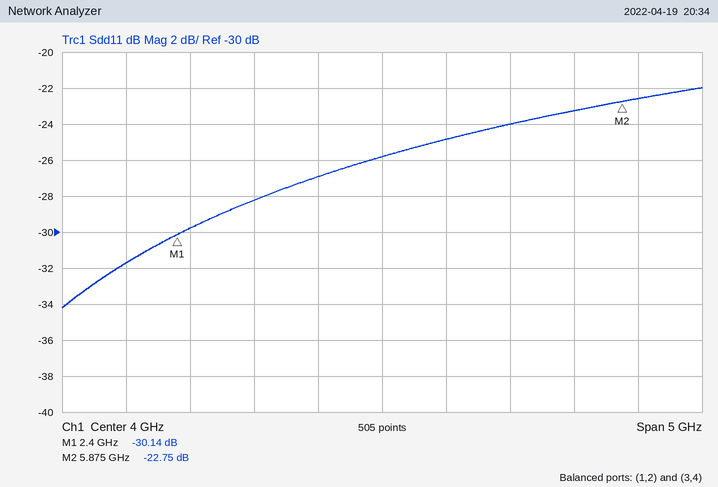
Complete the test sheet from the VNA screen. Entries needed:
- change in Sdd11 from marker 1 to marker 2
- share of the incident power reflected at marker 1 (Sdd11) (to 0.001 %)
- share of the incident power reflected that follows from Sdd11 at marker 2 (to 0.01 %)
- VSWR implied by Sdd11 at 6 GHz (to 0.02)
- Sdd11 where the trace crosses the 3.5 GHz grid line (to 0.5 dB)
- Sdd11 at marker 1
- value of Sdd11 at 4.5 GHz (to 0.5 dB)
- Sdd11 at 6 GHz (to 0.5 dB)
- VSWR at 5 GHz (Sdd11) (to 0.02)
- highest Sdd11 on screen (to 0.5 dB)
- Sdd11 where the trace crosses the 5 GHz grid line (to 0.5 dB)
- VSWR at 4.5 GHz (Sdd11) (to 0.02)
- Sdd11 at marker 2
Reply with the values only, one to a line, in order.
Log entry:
7.39 dB
0.097 %
0.53 %
1.16
-27.0 dB
-30.14 dB
-25.0 dB
-22.5 dB
1.14
-22.0 dB
-24.0 dB
1.12
-22.75 dB
